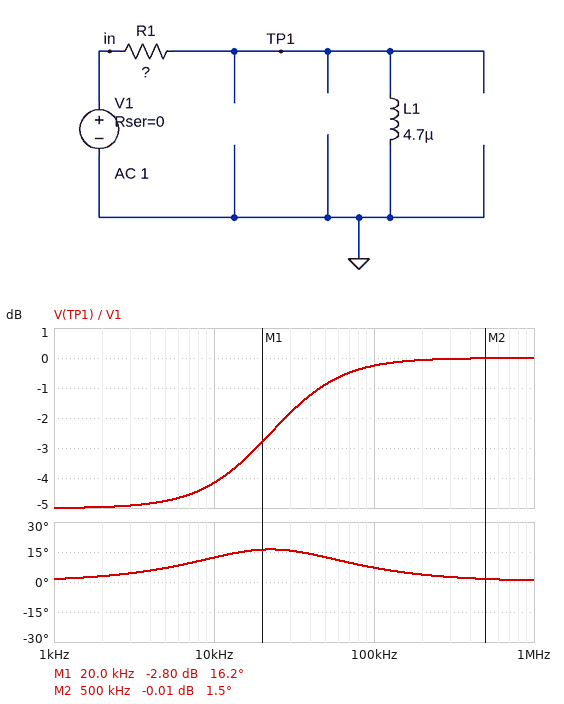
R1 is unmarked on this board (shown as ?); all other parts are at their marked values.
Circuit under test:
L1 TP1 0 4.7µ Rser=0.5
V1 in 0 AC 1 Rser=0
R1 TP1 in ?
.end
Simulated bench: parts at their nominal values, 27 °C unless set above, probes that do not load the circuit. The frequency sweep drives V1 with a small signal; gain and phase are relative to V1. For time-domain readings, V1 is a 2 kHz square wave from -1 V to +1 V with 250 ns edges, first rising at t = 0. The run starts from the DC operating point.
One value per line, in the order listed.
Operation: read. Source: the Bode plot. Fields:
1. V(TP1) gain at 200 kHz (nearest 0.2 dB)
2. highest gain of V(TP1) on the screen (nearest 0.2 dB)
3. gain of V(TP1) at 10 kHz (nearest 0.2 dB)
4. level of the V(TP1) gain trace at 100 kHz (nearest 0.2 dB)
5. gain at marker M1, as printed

0 dB
0 dB
-4.2 dB
-0.2 dB
-2.80 dB
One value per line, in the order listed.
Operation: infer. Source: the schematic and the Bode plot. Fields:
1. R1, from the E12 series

0.39 Ω
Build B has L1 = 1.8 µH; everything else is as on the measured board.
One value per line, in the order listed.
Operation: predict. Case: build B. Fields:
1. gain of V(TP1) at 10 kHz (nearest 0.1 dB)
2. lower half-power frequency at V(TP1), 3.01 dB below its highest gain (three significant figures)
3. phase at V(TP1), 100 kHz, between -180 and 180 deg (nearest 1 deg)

-4.9 dB
47.8 kHz
14 deg
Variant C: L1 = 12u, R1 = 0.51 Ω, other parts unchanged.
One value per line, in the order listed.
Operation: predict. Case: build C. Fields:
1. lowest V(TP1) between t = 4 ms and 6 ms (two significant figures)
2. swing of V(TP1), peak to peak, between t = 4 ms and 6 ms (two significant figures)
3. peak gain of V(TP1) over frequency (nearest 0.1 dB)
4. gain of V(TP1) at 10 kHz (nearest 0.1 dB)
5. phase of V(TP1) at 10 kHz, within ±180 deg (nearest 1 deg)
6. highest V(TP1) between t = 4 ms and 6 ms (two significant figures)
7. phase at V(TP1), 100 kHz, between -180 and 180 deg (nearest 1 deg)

-1.5 V
3.0 V
0 dB
-2.9 dB
20 deg
1.5 V
4 deg
